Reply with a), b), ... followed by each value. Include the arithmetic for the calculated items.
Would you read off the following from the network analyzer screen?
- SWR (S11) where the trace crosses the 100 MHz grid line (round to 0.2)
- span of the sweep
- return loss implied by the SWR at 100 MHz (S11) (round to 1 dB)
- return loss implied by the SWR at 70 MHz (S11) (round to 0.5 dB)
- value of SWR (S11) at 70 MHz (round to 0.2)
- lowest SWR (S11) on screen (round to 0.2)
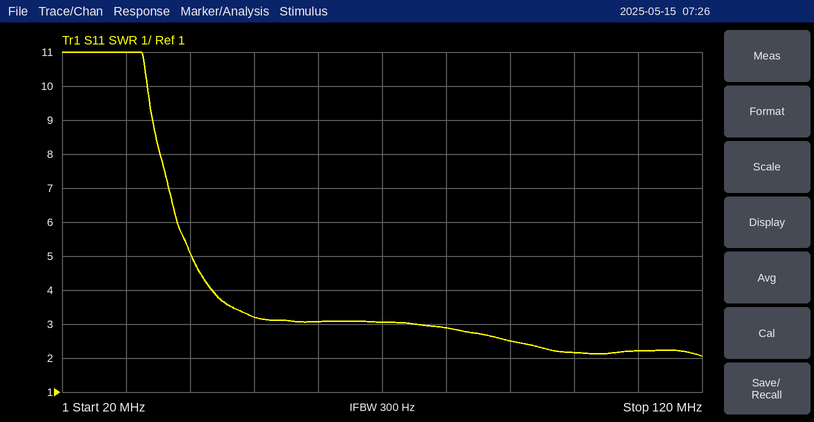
a) 2.2
b) 100 MHz
c) −20 log10((2.2 − 1)/(2.2 + 1)) ≈ 9 dB
d) −20 log10((3 − 1)/(3 + 1)) ≈ 6.0 dB
e) 3.0
f) 2.0
